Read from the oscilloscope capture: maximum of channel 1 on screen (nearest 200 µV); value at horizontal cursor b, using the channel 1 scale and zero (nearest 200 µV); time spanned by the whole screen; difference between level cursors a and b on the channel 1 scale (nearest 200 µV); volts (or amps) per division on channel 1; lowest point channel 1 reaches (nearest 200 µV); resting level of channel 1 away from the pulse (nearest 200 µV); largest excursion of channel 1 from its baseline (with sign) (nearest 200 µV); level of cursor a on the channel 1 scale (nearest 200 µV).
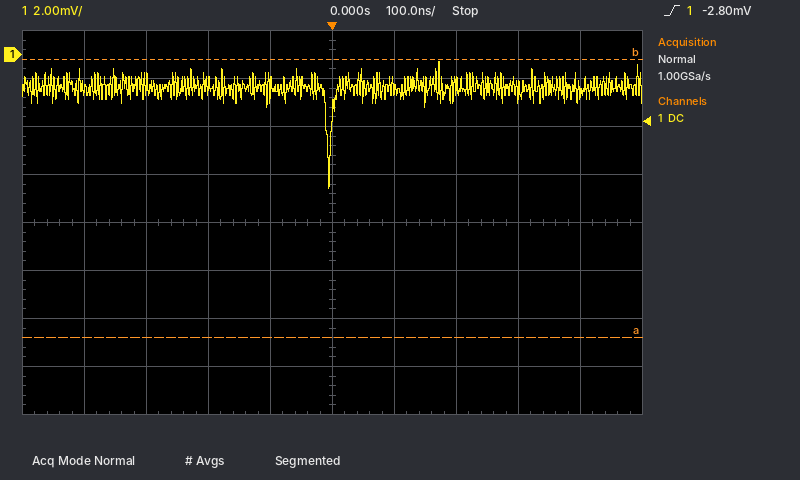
-200 µV
-200 µV
1 µs
11.6 mV
2 mV
-5.6 mV
-1.4 mV
-4.2 mV
-11.8 mV
